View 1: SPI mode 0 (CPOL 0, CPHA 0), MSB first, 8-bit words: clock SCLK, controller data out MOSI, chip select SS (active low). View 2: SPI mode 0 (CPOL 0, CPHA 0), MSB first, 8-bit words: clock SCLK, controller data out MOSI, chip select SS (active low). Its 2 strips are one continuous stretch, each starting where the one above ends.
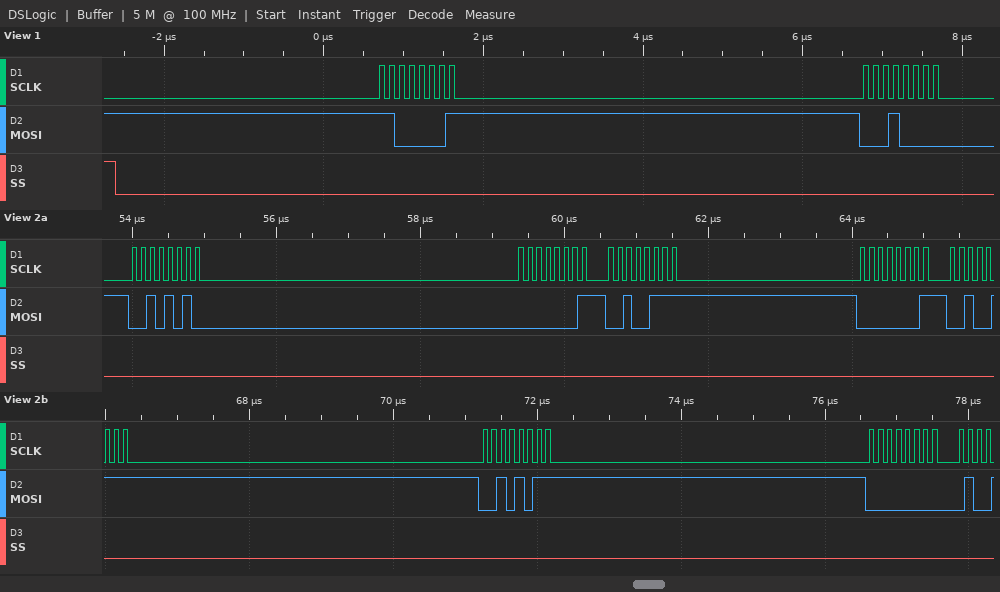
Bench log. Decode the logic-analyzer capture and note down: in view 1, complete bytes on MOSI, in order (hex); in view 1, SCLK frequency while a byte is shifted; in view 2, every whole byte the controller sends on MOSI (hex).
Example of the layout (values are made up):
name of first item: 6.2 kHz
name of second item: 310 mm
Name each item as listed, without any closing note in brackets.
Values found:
in view 1, complete bytes on MOSI, in order: C1 10
in view 1, SCLK frequency while a byte is shifted: 8 MHz
in view 2, every whole byte the controller sends on MOSI: 2A 01 27 01 27 2B 00
